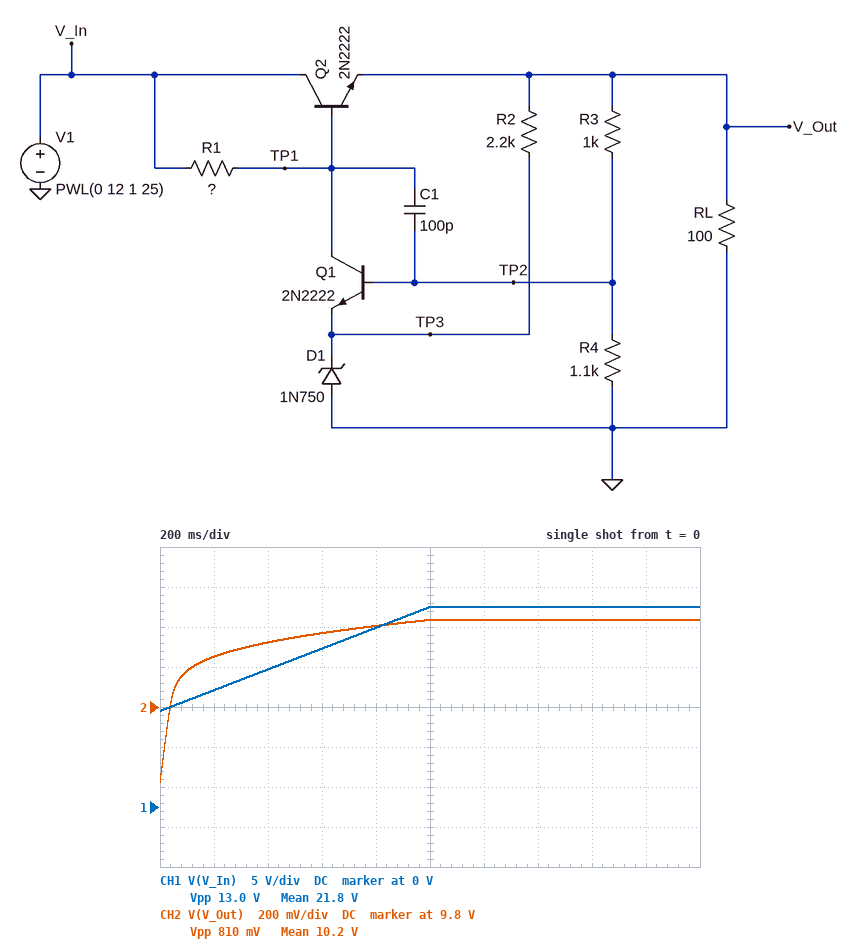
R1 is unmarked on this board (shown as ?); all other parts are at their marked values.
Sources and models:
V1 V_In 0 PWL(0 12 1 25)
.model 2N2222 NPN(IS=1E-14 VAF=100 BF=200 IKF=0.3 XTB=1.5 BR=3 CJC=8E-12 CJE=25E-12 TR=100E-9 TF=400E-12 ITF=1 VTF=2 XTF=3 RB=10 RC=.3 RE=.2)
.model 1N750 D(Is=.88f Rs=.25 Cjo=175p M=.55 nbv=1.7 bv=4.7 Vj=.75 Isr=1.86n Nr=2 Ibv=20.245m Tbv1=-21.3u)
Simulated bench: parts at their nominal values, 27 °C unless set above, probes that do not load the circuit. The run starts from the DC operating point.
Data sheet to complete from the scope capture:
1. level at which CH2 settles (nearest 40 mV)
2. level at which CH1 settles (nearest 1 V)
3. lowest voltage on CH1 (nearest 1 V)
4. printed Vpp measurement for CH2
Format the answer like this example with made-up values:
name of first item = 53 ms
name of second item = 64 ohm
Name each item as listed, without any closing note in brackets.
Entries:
level at which CH2 settles = 10.24 V
level at which CH1 settles = 25 V
lowest voltage on CH1 = 12 V
printed Vpp measurement for CH2 = 810 mV
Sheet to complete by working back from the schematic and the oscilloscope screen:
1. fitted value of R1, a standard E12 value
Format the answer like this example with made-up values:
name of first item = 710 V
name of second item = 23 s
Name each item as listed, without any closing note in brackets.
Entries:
fitted value of R1, a standard E12 value = 2.7 kΩ
